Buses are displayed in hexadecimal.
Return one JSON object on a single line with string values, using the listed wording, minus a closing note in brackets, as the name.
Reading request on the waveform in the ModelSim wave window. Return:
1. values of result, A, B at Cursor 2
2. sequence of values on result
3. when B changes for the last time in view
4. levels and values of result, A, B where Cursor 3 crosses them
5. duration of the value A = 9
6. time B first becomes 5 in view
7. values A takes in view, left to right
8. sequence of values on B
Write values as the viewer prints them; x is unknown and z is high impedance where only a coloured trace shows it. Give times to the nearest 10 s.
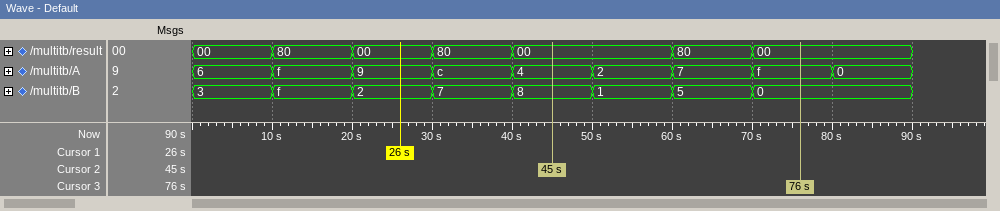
{"values of result, A, B at Cursor 2": "result=00, A=4, B=8", "sequence of values on result": "00, 80, 00, 80, 00, 80, 00", "when B changes for the last time in view": "70 s", "levels and values of result, A, B where Cursor 3 crosses them": "result=00, A=f, B=0", "duration of the value A = 9": "10 s", "time B first becomes 5 in view": "60 s", "values A takes in view, left to right": "6, f, 9, c, 4, 2, 7, f, 0", "sequence of values on B": "3, f, 2, 7, 8, 1, 5, 0"}
